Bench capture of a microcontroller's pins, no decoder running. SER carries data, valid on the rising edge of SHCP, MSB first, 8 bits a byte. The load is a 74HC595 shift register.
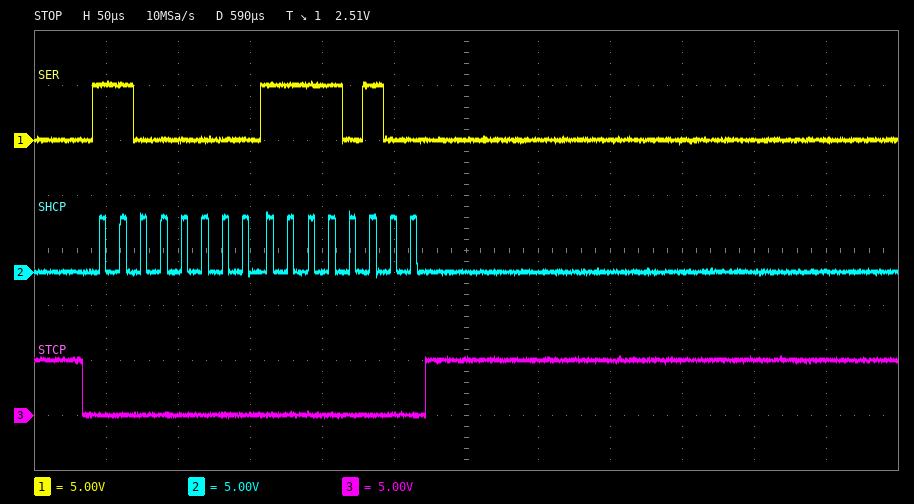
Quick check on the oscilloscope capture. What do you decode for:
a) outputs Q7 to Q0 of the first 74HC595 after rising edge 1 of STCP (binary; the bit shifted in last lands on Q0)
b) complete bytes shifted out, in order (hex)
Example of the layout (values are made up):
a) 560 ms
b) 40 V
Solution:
a) 11110100
b) 0xC0 0xF4
